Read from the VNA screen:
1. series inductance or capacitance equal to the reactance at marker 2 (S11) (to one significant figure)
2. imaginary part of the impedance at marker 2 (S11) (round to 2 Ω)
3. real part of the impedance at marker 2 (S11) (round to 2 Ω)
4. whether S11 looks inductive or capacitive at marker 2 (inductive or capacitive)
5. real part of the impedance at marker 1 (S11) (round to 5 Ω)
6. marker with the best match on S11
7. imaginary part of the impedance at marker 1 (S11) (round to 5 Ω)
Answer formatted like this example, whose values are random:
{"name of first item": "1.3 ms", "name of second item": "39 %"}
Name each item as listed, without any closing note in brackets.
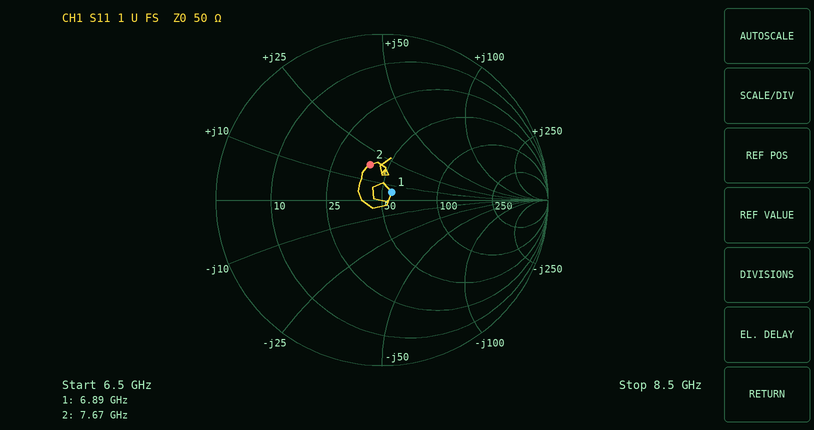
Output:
{"series inductance or capacitance equal to the reactance at marker 2 (S11)": "400 pH", "imaginary part of the impedance at marker 2 (S11)": "+18 Ω", "real part of the impedance at marker 2 (S11)": "40 Ω", "whether S11 looks inductive or capacitive at marker 2": "inductive", "real part of the impedance at marker 1 (S11)": "55 Ω", "marker with the best match on S11": "marker 1", "imaginary part of the impedance at marker 1 (S11)": "+5 Ω"}
